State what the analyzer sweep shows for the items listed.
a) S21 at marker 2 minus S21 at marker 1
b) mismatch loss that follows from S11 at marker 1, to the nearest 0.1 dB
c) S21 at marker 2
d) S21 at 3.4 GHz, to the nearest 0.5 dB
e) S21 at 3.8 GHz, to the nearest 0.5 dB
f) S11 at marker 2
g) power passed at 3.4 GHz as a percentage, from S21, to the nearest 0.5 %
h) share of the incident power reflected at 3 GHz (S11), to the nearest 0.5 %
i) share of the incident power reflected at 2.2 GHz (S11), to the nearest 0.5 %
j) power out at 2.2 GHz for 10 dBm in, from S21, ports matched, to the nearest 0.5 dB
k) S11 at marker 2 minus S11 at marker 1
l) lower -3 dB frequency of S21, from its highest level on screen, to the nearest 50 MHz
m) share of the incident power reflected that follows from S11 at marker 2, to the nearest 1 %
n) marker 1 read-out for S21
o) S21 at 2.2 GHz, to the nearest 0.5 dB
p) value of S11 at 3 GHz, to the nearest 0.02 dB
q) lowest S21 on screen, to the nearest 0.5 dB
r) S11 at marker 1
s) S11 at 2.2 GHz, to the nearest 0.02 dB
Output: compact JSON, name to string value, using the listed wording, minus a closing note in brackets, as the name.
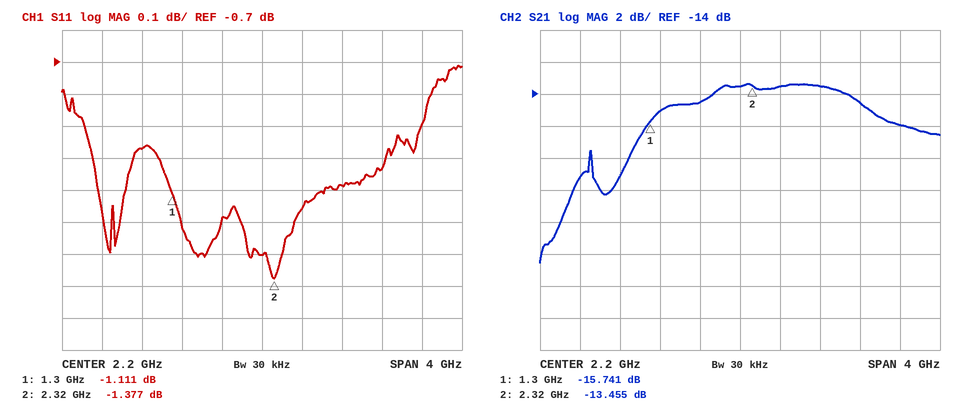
{"S21 at marker 2 minus S21 at marker 1": "2.286 dB", "mismatch loss that follows from S11 at marker 1, to the nearest 0.1 dB": "6.5 dB", "S21 at marker 2": "-13.455 dB", "S21 at 3.4 GHz, to the nearest 0.5 dB": "-14.5 dB", "S21 at 3.8 GHz, to the nearest 0.5 dB": "-16.0 dB", "S11 at marker 2": "-1.377 dB", "power passed at 3.4 GHz as a percentage, from S21, to the nearest 0.5 %": "3.5 %", "share of the incident power reflected at 3 GHz (S11), to the nearest 0.5 %": "78.0 %", "share of the incident power reflected at 2.2 GHz (S11), to the nearest 0.5 %": "74.0 %", "power out at 2.2 GHz for 10 dBm in, from S21, ports matched, to the nearest 0.5 dB": "-3.5 dBm", "S11 at marker 2 minus S11 at marker 1": "-0.266 dB", "lower -3 dB frequency of S21, from its highest level on screen, to the nearest 50 MHz": "1.25 GHz", "share of the incident power reflected that follows from S11 at marker 2, to the nearest 1 %": "73 %", "marker 1 read-out for S21": "-15.741 dB", "S21 at 2.2 GHz, to the nearest 0.5 dB": "-13.5 dB", "value of S11 at 3 GHz, to the nearest 0.02 dB": "-1.08 dB", "lowest S21 on screen, to the nearest 0.5 dB": "-24.5 dB", "S11 at marker 1": "-1.111 dB", "S11 at 2.2 GHz, to the nearest 0.02 dB": "-1.30 dB"}
